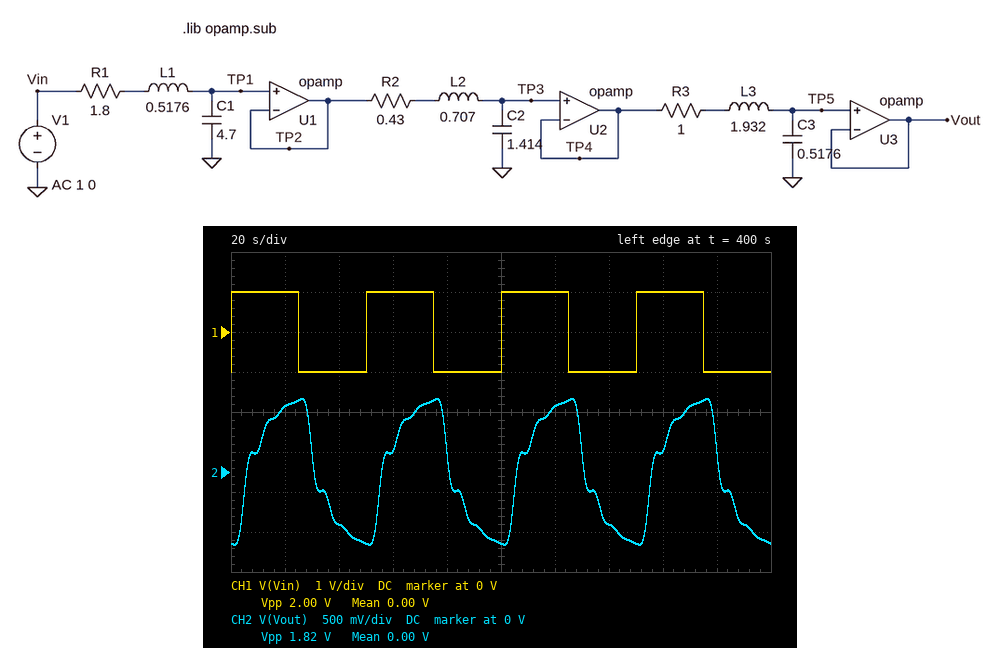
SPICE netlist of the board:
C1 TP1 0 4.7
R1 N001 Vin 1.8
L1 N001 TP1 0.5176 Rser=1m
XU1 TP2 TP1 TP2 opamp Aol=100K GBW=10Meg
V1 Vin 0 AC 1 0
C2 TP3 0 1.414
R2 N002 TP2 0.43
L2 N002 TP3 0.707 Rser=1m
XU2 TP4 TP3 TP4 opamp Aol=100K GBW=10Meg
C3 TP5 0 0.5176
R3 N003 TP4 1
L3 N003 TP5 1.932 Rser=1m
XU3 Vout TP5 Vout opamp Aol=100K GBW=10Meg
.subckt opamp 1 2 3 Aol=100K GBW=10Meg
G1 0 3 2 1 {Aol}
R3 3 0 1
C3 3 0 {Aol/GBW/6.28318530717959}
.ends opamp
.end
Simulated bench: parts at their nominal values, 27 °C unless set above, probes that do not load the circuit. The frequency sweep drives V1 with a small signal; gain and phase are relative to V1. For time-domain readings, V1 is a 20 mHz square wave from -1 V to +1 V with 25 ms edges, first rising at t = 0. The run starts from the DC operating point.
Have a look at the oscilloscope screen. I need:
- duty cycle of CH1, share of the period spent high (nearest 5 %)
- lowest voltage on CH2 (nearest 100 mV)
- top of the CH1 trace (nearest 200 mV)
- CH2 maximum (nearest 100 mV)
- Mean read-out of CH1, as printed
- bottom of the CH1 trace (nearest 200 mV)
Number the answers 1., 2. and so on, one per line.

1. 50 %
2. -900 mV
3. 1.0 V
4. 900 mV
5. 0.00 V
6. -1.0 V
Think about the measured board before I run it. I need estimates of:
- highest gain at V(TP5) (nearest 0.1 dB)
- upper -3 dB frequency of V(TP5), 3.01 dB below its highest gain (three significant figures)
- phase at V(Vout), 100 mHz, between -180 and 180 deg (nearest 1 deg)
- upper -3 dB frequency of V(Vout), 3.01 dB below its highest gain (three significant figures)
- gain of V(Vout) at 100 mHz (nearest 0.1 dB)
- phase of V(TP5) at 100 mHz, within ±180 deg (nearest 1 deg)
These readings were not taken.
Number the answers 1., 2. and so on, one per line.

1. 0 dB
2. 20.6 mHz
3. -150 deg
4. 20.6 mHz
5. -8.4 dB
6. -150 deg
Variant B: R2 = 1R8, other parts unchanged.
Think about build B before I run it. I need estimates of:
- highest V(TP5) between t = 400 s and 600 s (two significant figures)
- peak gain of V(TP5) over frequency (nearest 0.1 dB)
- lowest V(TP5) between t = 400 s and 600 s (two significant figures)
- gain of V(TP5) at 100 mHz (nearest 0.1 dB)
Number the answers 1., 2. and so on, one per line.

1. 880 mV
2. 0 dB
3. -880 mV
4. -15.9 dB
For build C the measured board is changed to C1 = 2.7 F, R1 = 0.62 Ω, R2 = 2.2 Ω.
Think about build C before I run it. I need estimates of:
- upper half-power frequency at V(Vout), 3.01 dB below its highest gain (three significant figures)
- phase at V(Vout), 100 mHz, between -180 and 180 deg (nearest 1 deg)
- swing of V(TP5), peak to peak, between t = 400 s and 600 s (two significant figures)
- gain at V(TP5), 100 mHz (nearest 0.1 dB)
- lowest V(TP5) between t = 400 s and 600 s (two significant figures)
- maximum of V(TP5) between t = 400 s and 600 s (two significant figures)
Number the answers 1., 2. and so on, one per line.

1. 74.3 mHz
2. -168 deg
3. 2.0 V
4. -4.1 dB
5. -1.0 V
6. 1.0 V
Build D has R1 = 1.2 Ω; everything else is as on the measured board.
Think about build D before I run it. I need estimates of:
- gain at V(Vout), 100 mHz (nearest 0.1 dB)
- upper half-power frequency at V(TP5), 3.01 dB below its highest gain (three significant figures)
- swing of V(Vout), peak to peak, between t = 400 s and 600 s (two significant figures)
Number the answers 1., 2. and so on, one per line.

1. -4.8 dB
2. 35.7 mHz
3. 2.0 V
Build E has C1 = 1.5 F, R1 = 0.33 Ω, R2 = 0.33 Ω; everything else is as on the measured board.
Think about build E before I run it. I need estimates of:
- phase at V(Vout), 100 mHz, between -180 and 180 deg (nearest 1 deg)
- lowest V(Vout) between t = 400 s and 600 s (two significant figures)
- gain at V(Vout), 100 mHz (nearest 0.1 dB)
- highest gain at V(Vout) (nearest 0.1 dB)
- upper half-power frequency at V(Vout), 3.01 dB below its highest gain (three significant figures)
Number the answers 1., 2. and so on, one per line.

1. -78 deg
2. -3.6 V
3. 9.1 dB
4. 17.9 dB
5. 174 mHz
